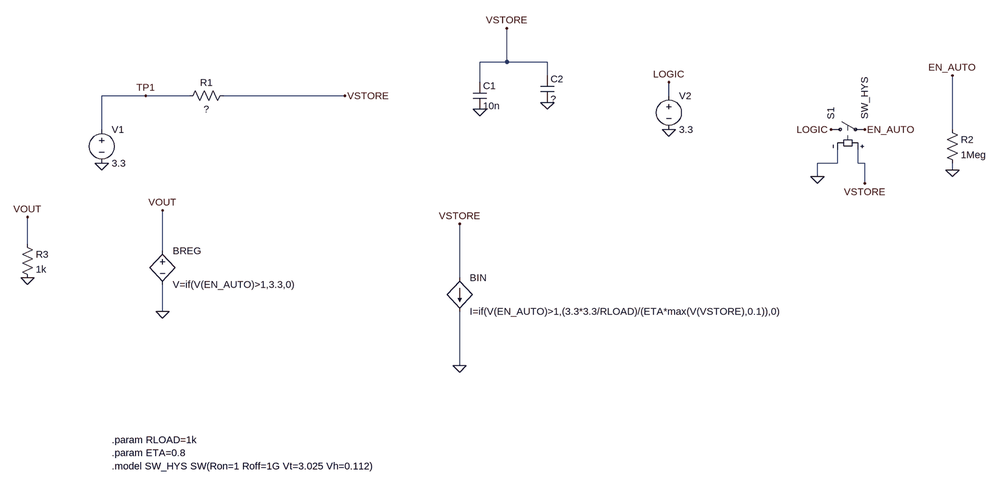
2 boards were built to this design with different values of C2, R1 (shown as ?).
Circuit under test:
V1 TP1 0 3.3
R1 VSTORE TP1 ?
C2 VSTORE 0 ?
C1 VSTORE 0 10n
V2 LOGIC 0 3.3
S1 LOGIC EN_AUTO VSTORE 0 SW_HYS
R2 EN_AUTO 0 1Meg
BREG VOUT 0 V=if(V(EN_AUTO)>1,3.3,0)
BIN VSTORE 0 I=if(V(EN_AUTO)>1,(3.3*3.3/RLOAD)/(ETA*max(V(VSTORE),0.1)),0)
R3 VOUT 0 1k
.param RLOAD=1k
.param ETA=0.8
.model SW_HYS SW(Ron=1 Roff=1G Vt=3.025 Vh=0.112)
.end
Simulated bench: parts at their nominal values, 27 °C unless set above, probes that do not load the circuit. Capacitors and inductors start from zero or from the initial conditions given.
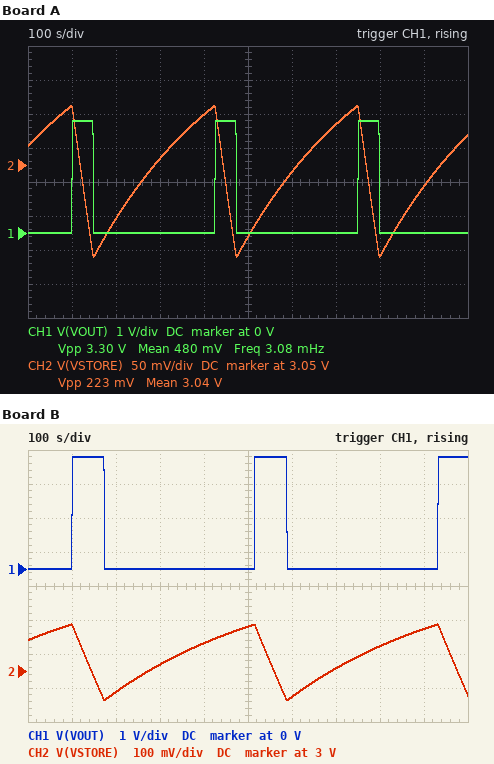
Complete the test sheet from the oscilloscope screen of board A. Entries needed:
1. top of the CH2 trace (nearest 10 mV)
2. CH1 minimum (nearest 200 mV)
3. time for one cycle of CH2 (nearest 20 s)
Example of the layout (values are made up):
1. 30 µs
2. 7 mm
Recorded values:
1. 3.14 V
2. 0 V
3. 320 s
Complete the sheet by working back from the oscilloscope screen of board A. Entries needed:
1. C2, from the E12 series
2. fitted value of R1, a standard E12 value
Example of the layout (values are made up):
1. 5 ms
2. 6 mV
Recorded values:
1. 820 mF
2. 390 Ω
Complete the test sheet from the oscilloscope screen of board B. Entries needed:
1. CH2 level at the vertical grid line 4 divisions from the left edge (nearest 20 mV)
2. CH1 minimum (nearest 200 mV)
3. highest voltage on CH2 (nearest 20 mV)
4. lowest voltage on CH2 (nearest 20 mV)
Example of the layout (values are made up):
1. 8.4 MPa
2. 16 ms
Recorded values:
1. 3.08 V
2. 0 V
3. 3.14 V
4. 2.92 V
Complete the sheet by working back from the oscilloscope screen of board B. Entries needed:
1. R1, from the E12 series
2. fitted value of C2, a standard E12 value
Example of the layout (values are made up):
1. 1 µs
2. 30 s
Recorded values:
1. 330 Ω
2. 1.2 F
